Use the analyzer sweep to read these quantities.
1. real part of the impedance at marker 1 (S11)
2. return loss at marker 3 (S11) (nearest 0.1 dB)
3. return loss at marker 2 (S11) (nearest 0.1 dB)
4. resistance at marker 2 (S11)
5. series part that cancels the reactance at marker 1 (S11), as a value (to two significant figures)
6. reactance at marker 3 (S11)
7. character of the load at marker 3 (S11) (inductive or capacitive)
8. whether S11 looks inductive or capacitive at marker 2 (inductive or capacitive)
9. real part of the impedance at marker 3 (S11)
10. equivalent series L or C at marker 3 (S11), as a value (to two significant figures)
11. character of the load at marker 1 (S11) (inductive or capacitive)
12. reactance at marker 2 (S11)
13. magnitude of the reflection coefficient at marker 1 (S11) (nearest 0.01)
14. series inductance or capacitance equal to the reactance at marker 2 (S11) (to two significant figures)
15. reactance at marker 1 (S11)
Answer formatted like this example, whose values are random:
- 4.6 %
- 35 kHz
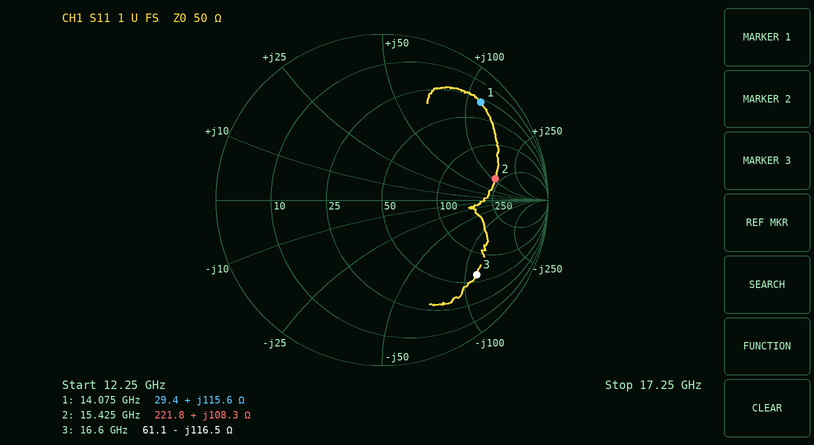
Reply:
- 29.4 Ω
- 2.8 dB
- 3.2 dB
- 221.8 Ω
- 98 fF
- -116.5 Ω
- capacitive
- inductive
- 61.1 Ω
- 82 fF
- inductive
- +108.3 Ω
- 0.84
- 1.1 nH
- +115.6 Ω
